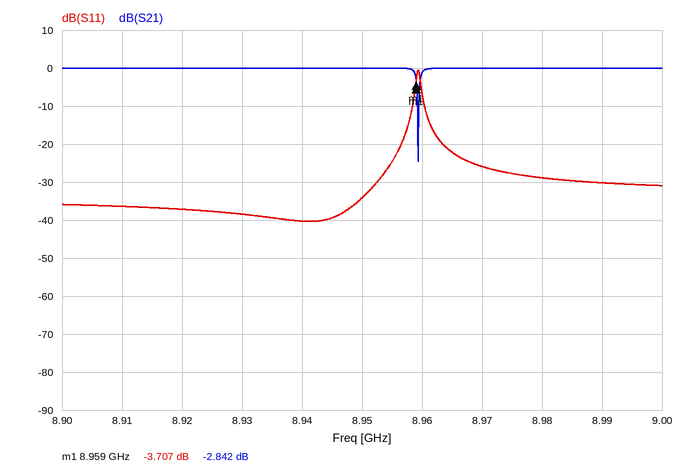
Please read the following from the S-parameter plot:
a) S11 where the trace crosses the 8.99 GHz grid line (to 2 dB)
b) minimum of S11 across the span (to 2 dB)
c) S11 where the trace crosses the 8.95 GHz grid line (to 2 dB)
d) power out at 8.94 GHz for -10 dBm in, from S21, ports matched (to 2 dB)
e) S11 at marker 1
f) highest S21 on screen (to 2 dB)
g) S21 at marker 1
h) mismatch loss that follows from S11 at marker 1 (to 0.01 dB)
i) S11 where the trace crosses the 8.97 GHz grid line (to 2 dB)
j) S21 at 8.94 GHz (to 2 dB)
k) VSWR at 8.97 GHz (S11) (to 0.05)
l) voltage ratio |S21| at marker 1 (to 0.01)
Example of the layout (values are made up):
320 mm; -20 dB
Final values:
-30 dB; -40 dB; -34 dB; -10 dBm; -3.707 dB; 0 dB; -2.842 dB; 2.41 dB; -26 dB; 0 dB; 1.10; 0.72
